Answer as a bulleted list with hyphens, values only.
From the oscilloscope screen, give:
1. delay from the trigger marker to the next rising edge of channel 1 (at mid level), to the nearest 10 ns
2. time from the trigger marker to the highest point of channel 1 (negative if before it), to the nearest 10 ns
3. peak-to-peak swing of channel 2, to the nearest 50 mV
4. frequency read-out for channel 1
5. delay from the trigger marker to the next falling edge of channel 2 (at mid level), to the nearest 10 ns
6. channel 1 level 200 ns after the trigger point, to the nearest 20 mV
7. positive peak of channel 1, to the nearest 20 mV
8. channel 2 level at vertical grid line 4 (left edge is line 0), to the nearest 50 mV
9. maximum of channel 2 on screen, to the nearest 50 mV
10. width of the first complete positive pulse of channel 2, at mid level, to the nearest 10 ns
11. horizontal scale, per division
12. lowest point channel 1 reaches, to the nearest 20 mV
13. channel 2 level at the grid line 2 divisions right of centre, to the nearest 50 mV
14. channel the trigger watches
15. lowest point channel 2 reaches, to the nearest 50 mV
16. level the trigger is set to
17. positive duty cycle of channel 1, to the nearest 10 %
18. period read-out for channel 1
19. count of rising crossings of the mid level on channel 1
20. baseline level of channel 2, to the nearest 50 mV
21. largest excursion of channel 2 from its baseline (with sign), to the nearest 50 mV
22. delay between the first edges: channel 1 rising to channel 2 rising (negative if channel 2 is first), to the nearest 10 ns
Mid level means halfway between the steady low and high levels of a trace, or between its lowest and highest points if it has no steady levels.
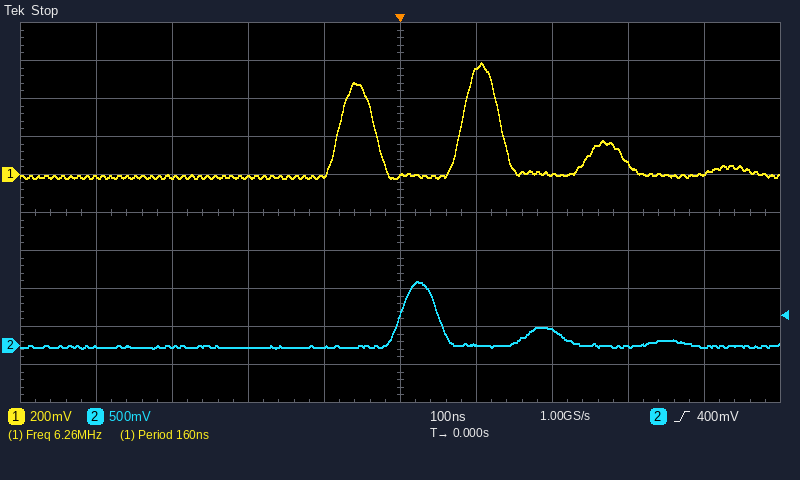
- 80 ns
- +110 ns
- 900 mV
- 6.26 MHz
- 50 ns
- 0 mV
- 580 mV
- 0 mV
- 850 mV
- 50 ns
- 100 ns
- -20 mV
- 200 mV
- channel 2
- -50 mV
- 400 mV
- 30 %
- 160 ns
- 2
- 0 mV
- +850 mV
- +80 ns
